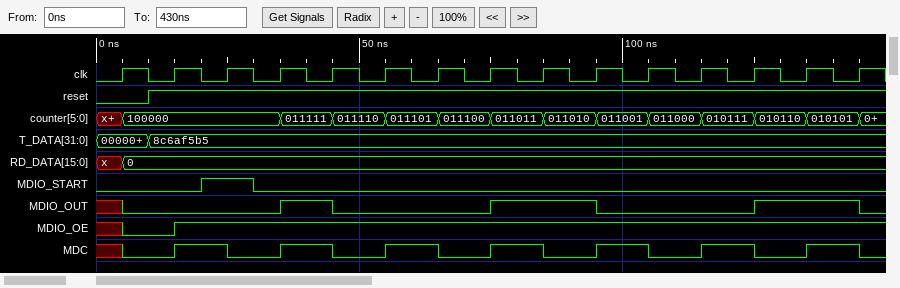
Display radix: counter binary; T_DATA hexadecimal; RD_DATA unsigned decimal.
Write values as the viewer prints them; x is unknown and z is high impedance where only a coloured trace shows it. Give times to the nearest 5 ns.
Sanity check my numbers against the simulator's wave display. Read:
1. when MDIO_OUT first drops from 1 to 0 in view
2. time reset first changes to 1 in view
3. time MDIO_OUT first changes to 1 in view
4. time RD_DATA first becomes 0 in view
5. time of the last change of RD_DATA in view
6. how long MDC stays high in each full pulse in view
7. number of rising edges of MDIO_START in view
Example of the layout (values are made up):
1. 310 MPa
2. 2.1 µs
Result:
1. 45 ns
2. 10 ns
3. 35 ns
4. 5 ns
5. 5 ns
6. 10 ns, 10 ns, 10 ns, 10 ns, 10 ns, 10 ns, 10 ns
7. 1
